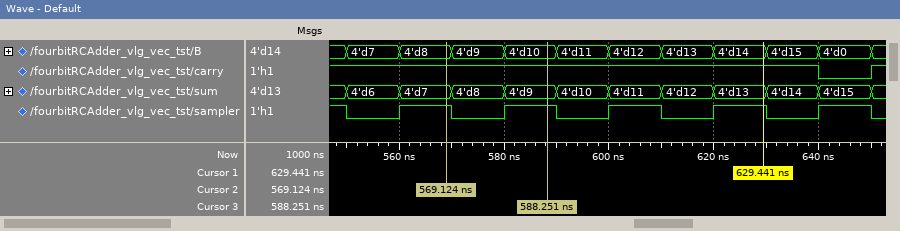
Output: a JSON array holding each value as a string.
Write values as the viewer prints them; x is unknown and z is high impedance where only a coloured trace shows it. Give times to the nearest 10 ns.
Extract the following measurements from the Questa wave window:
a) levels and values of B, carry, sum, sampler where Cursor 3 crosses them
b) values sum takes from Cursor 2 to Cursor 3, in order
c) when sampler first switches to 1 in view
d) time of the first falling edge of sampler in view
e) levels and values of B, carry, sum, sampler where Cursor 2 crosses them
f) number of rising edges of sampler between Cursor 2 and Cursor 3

["B=4'd10, carry=1, sum=4'd9, sampler=1", "4'd7, 4'd8, 4'd9", "560 ns", "550 ns", "B=4'd8, carry=1, sum=4'd7, sampler=1", "1"]
